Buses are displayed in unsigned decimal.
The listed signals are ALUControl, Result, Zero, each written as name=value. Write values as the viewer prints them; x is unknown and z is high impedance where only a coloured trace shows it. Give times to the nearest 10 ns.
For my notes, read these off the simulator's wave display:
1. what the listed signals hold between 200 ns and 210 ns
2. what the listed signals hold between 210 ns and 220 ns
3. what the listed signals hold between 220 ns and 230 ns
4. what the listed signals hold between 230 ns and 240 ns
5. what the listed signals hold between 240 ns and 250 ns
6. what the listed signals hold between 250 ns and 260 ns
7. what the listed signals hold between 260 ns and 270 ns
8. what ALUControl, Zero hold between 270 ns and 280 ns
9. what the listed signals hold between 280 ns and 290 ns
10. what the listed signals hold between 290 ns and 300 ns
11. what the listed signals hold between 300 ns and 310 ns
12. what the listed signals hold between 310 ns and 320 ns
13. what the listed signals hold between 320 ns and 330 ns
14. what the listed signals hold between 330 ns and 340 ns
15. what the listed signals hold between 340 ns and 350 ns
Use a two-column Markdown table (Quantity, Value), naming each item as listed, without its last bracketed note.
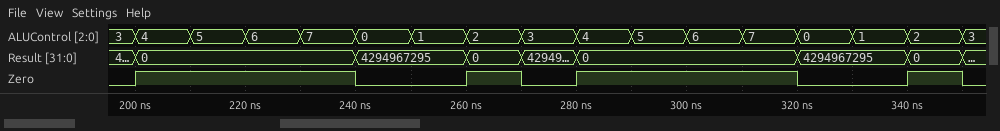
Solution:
| Quantity | Value |
|---|---|
| what the listed signals hold between 200 ns and 210 ns | ALUControl=4, Result=0, Zero=1 |
| what the listed signals hold between 210 ns and 220 ns | ALUControl=5, Result=0, Zero=1 |
| what the listed signals hold between 220 ns and 230 ns | ALUControl=6, Result=0, Zero=1 |
| what the listed signals hold between 230 ns and 240 ns | ALUControl=7, Result=0, Zero=1 |
| what the listed signals hold between 240 ns and 250 ns | ALUControl=0, Result=4294967295, Zero=0 |
| what the listed signals hold between 250 ns and 260 ns | ALUControl=1, Result=4294967295, Zero=0 |
| what the listed signals hold between 260 ns and 270 ns | ALUControl=2, Result=0, Zero=1 |
| what ALUControl, Zero hold between 270 ns and 280 ns | ALUControl=3, Zero=0 |
| what the listed signals hold between 280 ns and 290 ns | ALUControl=4, Result=0, Zero=1 |
| what the listed signals hold between 290 ns and 300 ns | ALUControl=5, Result=0, Zero=1 |
| what the listed signals hold between 300 ns and 310 ns | ALUControl=6, Result=0, Zero=1 |
| what the listed signals hold between 310 ns and 320 ns | ALUControl=7, Result=0, Zero=1 |
| what the listed signals hold between 320 ns and 330 ns | ALUControl=0, Result=4294967295, Zero=0 |
| what the listed signals hold between 330 ns and 340 ns | ALUControl=1, Result=4294967295, Zero=0 |
| what the listed signals hold between 340 ns and 350 ns | ALUControl=2, Result=0, Zero=1 |
